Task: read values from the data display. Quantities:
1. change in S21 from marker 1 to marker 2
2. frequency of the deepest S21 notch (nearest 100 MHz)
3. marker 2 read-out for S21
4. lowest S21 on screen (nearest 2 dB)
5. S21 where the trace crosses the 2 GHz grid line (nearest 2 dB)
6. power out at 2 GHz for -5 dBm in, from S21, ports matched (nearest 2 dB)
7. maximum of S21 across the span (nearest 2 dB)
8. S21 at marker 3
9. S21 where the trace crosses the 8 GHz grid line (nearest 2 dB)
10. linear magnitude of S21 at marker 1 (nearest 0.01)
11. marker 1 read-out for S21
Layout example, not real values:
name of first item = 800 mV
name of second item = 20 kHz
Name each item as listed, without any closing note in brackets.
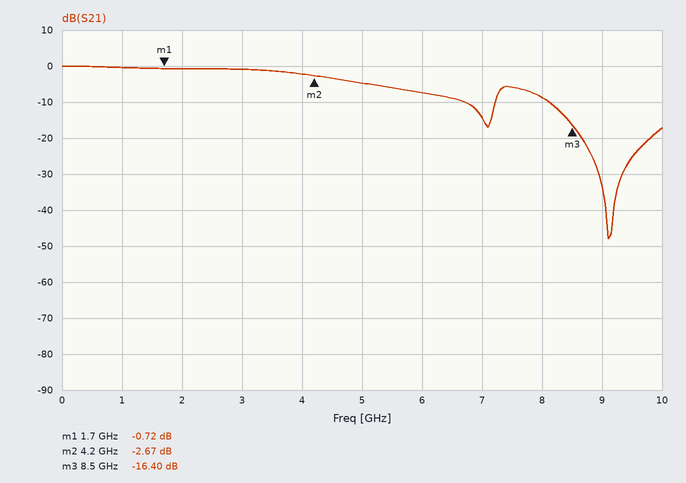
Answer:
change in S21 from marker 1 to marker 2 = -1.95 dB
frequency of the deepest S21 notch = 9.1 GHz
marker 2 read-out for S21 = -2.67 dB
lowest S21 on screen = -48 dB
S21 where the trace crosses the 2 GHz grid line = 0 dB
power out at 2 GHz for -5 dBm in, from S21, ports matched = -6 dBm
maximum of S21 across the span = 0 dB
S21 at marker 3 = -16.40 dB
S21 where the trace crosses the 8 GHz grid line = -8 dB
linear magnitude of S21 at marker 1 = 0.92
marker 1 read-out for S21 = -0.72 dB
